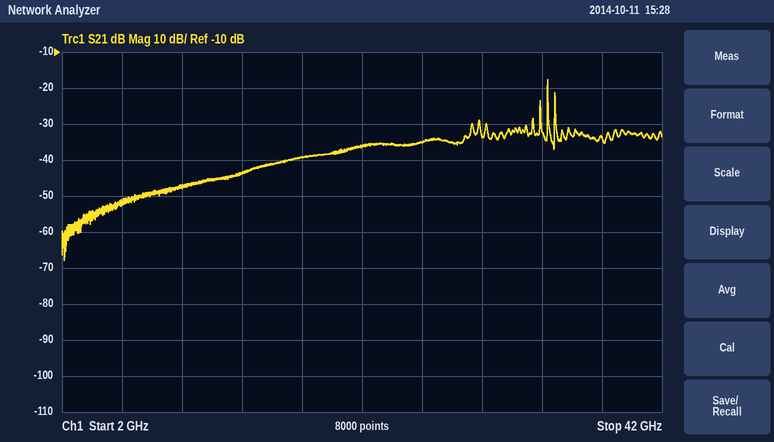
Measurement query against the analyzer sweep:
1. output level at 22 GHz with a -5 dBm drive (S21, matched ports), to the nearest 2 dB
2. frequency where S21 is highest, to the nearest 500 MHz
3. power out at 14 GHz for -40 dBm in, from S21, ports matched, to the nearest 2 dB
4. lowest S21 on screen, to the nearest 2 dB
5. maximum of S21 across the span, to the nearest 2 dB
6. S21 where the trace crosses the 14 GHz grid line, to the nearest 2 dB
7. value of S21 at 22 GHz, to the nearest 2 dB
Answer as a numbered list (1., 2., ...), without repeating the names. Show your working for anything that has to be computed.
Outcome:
1. -5 dBm + (-36 dB) = -42 dBm
2. 34.5 GHz
3. -40 dBm + (-44 dB) = -84 dBm
4. -68 dB
5. -18 dB
6. -44 dB
7. -36 dB
